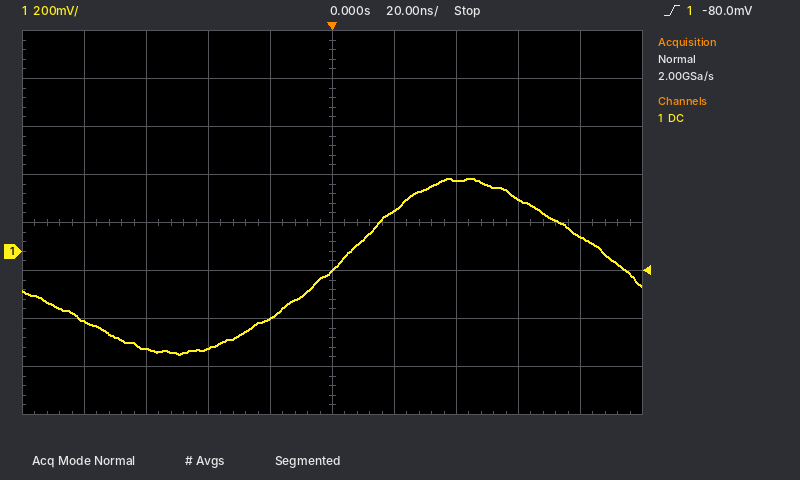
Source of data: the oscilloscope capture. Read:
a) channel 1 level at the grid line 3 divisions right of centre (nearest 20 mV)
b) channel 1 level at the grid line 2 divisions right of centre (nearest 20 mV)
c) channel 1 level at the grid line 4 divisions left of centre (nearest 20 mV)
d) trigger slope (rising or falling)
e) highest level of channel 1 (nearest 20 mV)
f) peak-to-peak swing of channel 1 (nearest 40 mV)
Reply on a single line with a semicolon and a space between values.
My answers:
220 mV; 300 mV; -300 mV; rising; 300 mV; 720 mV
